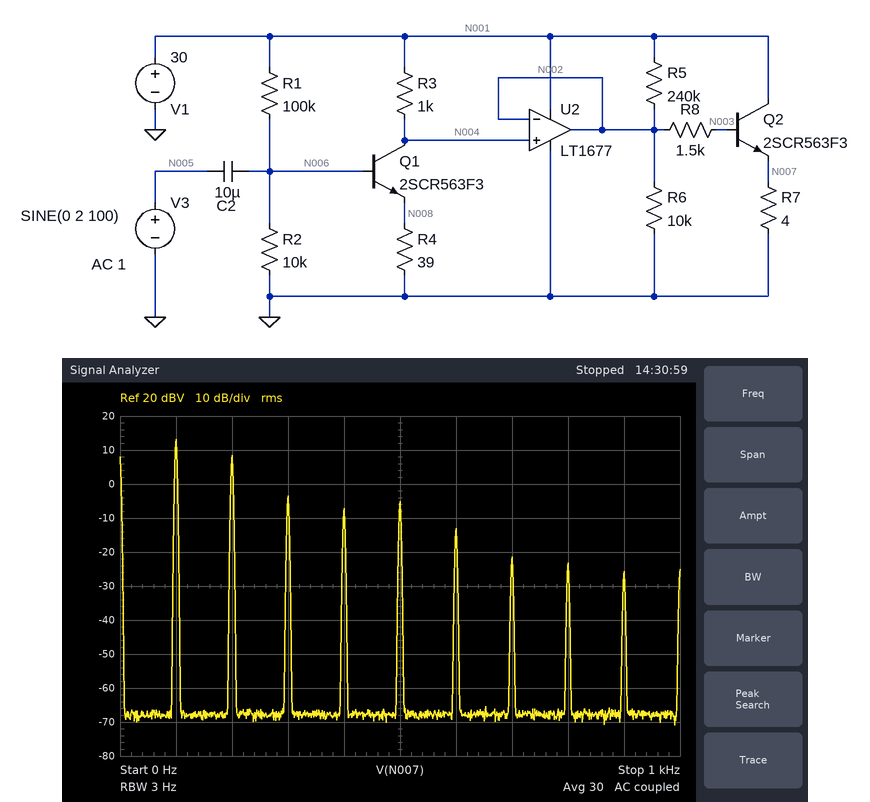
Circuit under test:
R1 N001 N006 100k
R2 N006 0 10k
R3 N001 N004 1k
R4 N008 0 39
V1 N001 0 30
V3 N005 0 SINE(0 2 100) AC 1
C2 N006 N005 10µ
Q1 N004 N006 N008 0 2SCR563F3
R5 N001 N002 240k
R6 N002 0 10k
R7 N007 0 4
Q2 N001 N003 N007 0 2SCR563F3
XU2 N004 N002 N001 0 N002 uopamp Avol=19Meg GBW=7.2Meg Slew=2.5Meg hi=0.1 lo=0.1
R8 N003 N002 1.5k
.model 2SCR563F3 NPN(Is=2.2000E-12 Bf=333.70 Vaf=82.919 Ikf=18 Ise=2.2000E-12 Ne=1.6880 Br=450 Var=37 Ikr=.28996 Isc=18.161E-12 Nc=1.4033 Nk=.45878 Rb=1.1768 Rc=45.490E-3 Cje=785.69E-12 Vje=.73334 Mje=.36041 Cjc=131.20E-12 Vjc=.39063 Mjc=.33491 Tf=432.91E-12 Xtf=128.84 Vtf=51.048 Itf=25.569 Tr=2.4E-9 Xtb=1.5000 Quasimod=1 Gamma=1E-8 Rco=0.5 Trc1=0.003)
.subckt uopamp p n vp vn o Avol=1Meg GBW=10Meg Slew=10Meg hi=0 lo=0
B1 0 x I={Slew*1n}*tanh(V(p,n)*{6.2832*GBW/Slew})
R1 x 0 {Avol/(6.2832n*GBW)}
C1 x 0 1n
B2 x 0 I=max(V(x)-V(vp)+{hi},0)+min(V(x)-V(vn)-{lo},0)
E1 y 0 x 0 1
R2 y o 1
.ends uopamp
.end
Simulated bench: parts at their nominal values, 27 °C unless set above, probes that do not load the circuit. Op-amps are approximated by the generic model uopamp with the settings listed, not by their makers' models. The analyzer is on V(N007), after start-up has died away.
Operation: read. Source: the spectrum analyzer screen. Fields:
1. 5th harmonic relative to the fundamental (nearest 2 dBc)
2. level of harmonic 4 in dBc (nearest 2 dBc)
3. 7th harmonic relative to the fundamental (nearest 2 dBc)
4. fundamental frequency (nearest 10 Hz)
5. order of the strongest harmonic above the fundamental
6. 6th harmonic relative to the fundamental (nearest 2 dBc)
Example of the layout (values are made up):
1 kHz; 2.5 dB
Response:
-18 dBc; -20 dBc; -34 dBc; 100 Hz; 2; -26 dBc
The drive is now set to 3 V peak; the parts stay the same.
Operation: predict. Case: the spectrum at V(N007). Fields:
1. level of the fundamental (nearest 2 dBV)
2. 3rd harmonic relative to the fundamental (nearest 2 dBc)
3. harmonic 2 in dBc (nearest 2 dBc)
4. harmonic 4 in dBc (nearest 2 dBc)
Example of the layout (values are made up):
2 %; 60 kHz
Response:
12 dBV; -10 dBc; -4 dBc; -30 dBc
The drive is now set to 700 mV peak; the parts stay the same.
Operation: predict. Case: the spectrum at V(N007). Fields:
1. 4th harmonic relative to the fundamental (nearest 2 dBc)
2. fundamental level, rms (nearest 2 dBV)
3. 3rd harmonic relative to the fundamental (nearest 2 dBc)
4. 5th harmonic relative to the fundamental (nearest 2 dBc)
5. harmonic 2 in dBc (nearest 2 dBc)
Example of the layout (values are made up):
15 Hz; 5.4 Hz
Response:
-36 dBc; 14 dBV; -26 dBc; -32 dBc; -26 dBc
